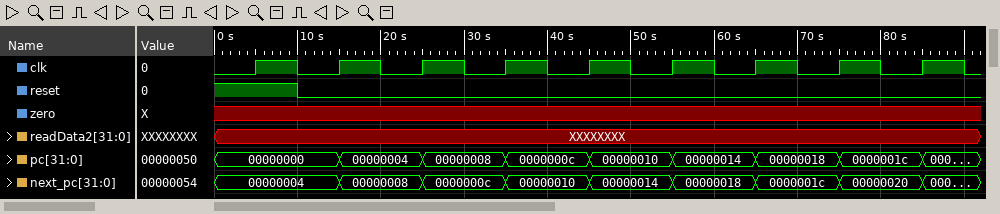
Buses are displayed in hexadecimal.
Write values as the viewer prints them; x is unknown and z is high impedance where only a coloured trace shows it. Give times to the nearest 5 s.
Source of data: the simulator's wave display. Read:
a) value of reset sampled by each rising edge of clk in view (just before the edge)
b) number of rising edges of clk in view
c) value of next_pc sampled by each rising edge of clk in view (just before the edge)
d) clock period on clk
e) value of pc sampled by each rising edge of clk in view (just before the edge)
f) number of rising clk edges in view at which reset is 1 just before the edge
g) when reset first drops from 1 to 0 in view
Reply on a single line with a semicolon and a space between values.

1 0 0 0 0 0 0 0 0; 9; 00000004, 00000004, 00000008, 0000000c, 00000010, 00000014, 00000018, 0000001c, 00000020; 10 s; 00000000, 00000000, 00000004, 00000008, 0000000c, 00000010, 00000014, 00000018, 0000001c; 1; 10 s
